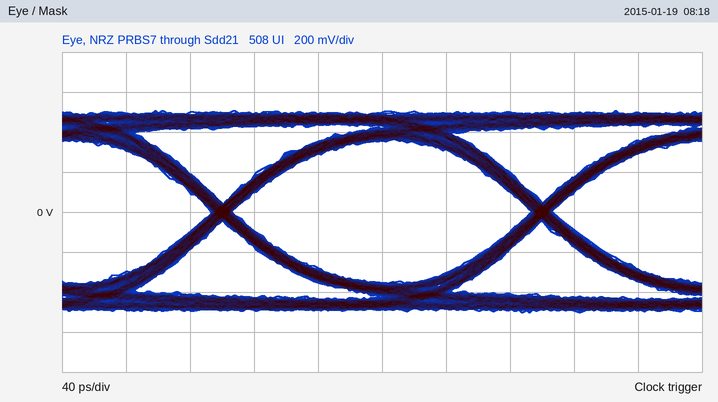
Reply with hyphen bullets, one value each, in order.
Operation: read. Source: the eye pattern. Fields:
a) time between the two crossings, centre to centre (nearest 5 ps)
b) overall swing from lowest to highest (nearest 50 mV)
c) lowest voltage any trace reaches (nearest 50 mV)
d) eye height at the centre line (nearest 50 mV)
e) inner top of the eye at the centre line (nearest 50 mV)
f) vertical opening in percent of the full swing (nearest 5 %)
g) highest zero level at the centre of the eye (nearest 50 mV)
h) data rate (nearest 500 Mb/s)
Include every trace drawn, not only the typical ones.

- 200 ps
- 1.00 V
- -500 mV
- 700 mV
- 350 mV
- 70 %
- -350 mV
- 5.0 Gb/s
